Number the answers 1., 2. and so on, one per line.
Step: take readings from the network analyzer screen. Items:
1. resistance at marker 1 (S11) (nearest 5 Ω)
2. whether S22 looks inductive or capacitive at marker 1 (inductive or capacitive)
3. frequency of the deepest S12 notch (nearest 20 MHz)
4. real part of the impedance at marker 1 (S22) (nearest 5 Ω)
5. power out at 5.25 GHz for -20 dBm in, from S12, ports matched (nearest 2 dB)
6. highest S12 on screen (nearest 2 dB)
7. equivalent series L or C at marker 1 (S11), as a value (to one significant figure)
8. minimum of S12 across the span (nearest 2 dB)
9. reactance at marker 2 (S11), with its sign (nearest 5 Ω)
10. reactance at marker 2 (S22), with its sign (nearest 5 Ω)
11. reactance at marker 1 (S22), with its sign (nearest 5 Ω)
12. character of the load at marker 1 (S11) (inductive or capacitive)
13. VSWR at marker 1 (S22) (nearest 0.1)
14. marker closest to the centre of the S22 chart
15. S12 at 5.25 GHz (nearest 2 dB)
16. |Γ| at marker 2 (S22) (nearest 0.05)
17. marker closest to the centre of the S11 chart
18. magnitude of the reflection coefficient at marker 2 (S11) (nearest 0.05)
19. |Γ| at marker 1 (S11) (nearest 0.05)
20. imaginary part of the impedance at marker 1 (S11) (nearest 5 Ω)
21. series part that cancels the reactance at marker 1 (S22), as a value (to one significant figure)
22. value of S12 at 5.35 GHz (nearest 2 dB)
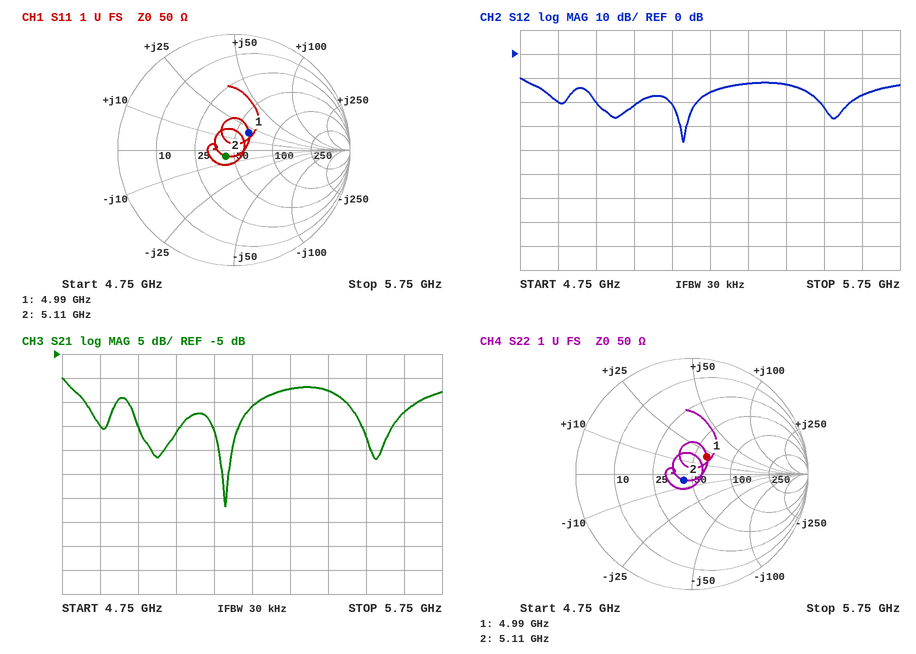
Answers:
1. 60 Ω
2. inductive
3. 5.18 GHz
4. 60 Ω
5. -36 dBm
6. -10 dB
7. 600 pH
8. -36 dB
9. -5 Ω
10. -5 Ω
11. +20 Ω
12. inductive
13. 1.5
14. marker 2
15. -16 dB
16. 0.10
17. marker 2
18. 0.10
19. 0.20
20. +20 Ω
21. 2 pF
22. -12 dB
